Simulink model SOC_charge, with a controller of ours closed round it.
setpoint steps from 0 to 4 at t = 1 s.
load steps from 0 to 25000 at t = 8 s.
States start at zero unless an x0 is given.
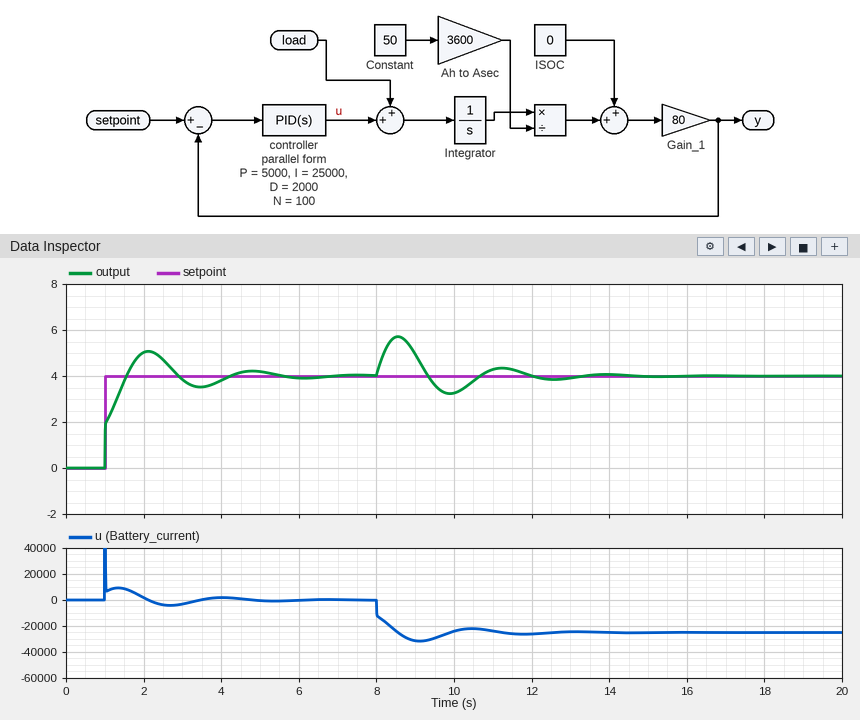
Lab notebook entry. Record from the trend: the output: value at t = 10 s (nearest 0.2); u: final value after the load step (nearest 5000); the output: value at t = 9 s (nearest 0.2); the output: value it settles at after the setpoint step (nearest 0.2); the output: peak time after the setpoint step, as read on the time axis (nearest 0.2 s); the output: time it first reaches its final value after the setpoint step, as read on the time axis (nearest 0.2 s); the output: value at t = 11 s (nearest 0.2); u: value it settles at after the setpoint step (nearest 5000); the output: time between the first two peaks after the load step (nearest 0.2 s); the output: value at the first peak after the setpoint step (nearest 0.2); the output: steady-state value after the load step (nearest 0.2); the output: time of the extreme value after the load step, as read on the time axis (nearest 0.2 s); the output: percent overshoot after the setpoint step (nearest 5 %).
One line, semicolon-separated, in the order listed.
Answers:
3.2; -25000; 5.0; 4.0; 2.2 s; 1.6 s; 4.2; 0; 2.6 s; 5.0; 4.0; 8.6 s; 25 %
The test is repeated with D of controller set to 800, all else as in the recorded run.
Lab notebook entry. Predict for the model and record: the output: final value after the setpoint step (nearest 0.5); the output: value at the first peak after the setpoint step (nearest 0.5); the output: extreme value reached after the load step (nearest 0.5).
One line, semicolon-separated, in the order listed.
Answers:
4.0; 5.5; 6.0
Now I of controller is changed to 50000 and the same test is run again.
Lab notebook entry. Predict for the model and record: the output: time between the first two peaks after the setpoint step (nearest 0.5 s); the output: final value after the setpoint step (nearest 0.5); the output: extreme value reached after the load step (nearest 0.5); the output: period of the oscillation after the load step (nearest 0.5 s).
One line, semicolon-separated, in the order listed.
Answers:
2.0 s; 4.0; 5.5; 2.0 s
